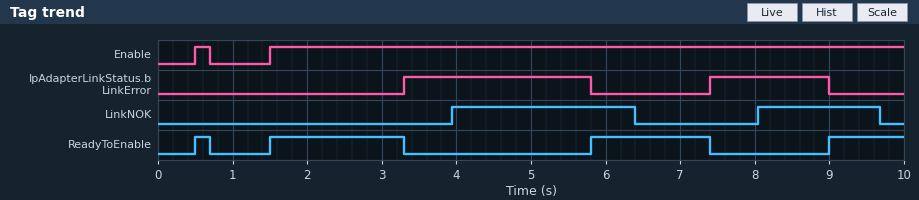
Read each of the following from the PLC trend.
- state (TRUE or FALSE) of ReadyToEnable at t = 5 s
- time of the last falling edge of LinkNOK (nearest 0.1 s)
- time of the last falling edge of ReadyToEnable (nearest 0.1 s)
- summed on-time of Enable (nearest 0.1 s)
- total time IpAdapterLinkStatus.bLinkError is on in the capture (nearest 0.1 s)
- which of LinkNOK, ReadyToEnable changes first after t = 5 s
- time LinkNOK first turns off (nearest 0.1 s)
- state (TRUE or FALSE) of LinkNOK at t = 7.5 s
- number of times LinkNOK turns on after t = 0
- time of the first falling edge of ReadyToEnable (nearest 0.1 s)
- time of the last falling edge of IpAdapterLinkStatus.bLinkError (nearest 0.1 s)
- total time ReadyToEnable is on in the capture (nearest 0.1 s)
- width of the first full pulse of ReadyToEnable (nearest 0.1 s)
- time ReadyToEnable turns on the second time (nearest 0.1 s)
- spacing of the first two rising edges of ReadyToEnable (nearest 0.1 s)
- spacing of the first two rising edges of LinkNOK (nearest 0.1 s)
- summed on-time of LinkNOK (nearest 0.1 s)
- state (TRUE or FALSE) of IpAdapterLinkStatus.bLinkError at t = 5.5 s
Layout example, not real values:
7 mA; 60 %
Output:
FALSE; 9.7 s; 7.4 s; 8.7 s; 4.1 s; ReadyToEnable; 6.4 s; FALSE; 2; 0.7 s; 9.0 s; 4.6 s; 0.2 s; 1.5 s; 1.0 s; 4.1 s; 4.1 s; TRUE
